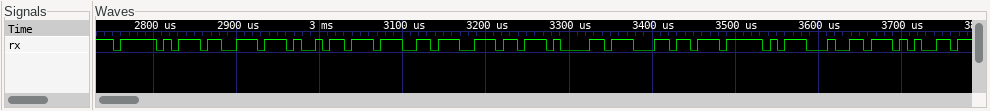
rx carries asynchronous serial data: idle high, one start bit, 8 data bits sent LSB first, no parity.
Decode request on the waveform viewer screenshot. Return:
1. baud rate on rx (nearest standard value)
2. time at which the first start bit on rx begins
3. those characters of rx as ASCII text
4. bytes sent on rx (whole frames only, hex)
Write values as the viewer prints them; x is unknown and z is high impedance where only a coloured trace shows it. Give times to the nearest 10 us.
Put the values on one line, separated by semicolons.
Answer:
115200 baud; 2750 us; "_signal_de"; 5F, 73, 69, 67, 6E, 61, 6C, 5F, 64, 65
